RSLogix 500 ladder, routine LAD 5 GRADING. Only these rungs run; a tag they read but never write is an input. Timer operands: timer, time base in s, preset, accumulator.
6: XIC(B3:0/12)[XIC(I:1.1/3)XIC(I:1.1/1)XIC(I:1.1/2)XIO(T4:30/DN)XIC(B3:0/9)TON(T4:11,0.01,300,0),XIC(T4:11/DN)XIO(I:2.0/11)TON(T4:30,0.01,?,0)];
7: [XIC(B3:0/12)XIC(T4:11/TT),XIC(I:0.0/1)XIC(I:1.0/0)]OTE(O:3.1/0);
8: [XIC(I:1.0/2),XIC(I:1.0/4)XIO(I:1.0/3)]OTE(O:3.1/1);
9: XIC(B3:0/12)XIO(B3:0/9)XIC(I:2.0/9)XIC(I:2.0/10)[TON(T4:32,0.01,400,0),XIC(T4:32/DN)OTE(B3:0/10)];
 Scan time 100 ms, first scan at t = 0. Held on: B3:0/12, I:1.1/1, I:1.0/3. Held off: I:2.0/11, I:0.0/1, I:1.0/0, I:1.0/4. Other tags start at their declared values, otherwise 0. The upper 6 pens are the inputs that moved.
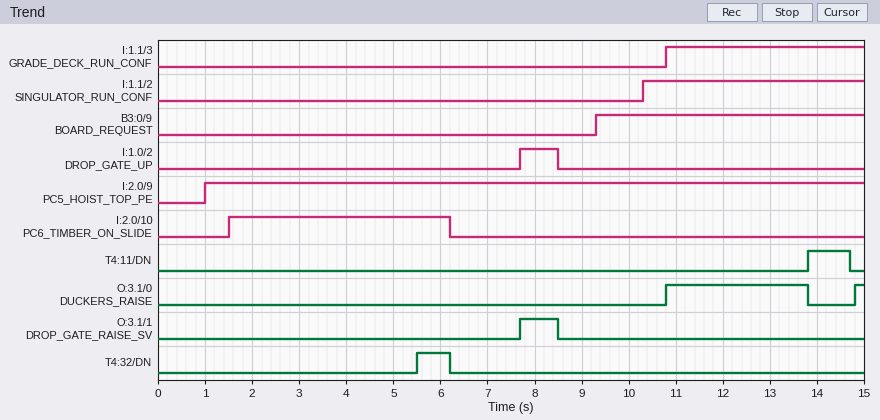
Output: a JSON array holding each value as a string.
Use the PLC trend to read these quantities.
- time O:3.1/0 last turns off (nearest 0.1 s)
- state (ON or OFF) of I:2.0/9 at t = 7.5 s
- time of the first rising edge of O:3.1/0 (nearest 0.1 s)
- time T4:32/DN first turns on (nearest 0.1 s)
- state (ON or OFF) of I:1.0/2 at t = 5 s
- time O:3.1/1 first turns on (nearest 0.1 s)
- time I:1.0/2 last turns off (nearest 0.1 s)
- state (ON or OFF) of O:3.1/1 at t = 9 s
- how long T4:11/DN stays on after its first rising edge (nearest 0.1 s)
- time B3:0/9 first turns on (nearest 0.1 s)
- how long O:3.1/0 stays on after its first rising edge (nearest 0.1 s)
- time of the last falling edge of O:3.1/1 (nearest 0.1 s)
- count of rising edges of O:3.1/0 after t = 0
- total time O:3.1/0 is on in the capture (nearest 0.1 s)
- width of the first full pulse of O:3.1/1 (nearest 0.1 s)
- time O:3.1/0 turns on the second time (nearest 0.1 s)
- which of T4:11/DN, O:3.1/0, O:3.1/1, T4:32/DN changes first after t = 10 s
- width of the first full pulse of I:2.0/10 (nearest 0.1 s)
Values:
["13.8 s", "ON", "10.8 s", "5.5 s", "OFF", "7.7 s", "8.5 s", "OFF", "0.9 s", "9.3 s", "3.0 s", "8.5 s", "2", "3.2 s", "0.8 s", "14.8 s", "O:3.1/0", "4.7 s"]
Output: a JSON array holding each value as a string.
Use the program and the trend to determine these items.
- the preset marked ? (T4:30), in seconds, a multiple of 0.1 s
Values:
["0.8 s"]
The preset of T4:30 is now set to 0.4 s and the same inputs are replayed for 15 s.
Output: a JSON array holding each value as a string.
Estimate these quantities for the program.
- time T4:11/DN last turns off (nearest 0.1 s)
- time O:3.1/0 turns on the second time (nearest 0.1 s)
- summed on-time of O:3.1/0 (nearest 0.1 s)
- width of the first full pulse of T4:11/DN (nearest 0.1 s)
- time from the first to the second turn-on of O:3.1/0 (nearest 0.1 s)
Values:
["14.3 s", "14.4 s", "3.6 s", "0.5 s", "3.6 s"]
